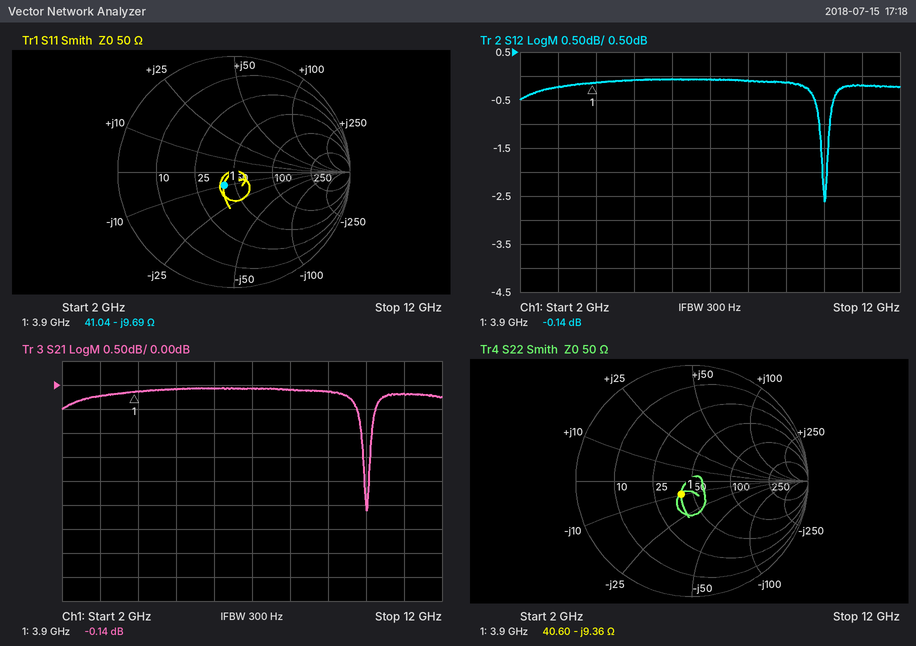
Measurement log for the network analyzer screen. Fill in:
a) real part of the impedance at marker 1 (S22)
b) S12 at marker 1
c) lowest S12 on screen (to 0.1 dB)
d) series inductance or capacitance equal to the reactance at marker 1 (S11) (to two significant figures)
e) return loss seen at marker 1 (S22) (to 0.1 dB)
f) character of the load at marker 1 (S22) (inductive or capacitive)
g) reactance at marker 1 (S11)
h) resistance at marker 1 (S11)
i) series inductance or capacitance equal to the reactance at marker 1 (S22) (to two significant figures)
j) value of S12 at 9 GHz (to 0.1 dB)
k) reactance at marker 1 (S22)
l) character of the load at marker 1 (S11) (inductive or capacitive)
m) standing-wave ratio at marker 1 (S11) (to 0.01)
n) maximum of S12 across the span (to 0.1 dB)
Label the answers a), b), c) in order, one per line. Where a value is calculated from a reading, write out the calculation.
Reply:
a) 40.60 Ω
b) -0.14 dB
c) -2.6 dB
d) C = 1/(2π × 3.9 GHz × 9.69 Ω) ≈ 4.2 pF
e) 16.7 dB
f) capacitive
g) -9.69 Ω
h) 41.04 Ω
i) C = 1/(2π × 3.9 GHz × 9.36 Ω) ≈ 4.4 pF
j) -0.1 dB
k) -9.36 Ω
l) capacitive
m) 1.34
n) -0.1 dB
